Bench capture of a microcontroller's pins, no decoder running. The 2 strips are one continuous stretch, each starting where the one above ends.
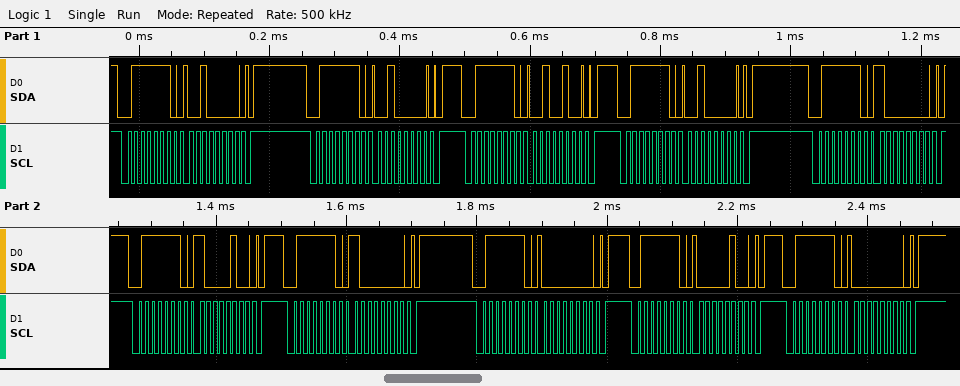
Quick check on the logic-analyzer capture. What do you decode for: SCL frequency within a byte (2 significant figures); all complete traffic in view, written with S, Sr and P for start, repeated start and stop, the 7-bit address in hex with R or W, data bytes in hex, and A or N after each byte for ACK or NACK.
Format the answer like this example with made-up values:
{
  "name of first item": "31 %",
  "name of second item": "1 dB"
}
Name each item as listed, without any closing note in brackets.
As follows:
{
  "SCL frequency within a byte": "100 kHz",
  "all complete traffic in view, written with S, Sr and P for start, repeated start and stop, the 7-bit address in hex with R or W, data bytes in hex, and A or N after each byte for ACK or NACK": "S 3FW A 20 A P S 3FW A 20 A P S 3FW A 24 A P S 3FW A 20 A P S 3FW A 80 A P S 3FW A 84 A P S 3FW A 80 A P S 3FW A 00 A P S 3FW A 04 A P S 3FW A 00 A P"
}
